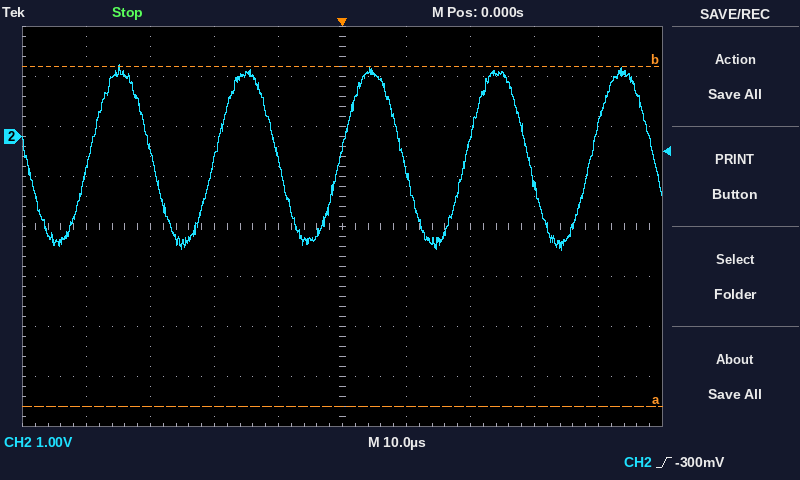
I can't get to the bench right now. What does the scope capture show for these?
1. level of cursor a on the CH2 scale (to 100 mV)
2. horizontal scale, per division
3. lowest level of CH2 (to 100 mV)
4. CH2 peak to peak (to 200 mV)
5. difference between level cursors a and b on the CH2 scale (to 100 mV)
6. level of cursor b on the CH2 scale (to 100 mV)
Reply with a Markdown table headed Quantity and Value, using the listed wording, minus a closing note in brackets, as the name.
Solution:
| Quantity | Value |
|---|---|
| level of cursor a on the CH2 scale | -5.4 V |
| horizontal scale, per division | 10 µs |
| lowest level of CH2 | -2.3 V |
| CH2 peak to peak | 3.8 V |
| difference between level cursors a and b on the CH2 scale | 6.8 V |
| level of cursor b on the CH2 scale | 1.4 V |
